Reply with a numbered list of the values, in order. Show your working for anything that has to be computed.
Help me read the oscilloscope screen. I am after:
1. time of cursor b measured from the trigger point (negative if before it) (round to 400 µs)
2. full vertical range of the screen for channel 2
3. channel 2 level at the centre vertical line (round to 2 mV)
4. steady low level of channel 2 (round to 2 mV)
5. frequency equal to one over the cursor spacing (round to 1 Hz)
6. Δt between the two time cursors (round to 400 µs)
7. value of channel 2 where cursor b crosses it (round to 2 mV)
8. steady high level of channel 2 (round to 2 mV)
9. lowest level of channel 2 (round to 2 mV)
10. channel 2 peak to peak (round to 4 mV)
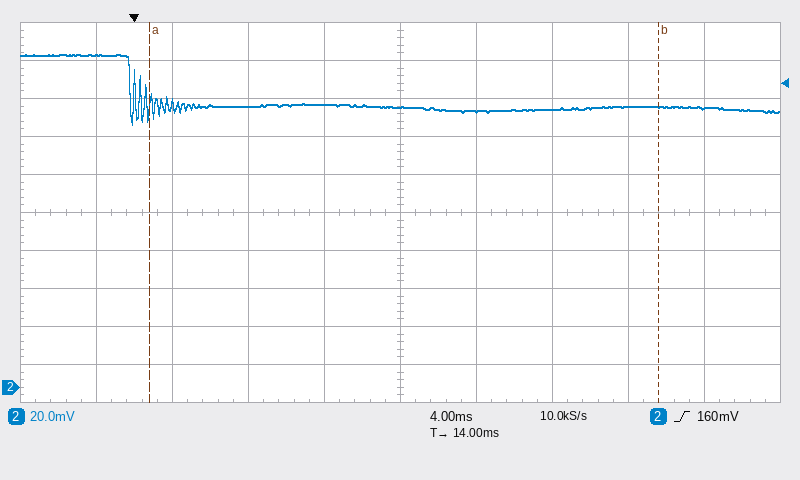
1. +27.6 ms
2. 200 mV
3. 148 mV
4. 148 mV
5. 1 / 26.8 ms ≈ 37 Hz
6. 26.8 ms
7. 148 mV
8. 174 mV
9. 138 mV
10. 36 mV
